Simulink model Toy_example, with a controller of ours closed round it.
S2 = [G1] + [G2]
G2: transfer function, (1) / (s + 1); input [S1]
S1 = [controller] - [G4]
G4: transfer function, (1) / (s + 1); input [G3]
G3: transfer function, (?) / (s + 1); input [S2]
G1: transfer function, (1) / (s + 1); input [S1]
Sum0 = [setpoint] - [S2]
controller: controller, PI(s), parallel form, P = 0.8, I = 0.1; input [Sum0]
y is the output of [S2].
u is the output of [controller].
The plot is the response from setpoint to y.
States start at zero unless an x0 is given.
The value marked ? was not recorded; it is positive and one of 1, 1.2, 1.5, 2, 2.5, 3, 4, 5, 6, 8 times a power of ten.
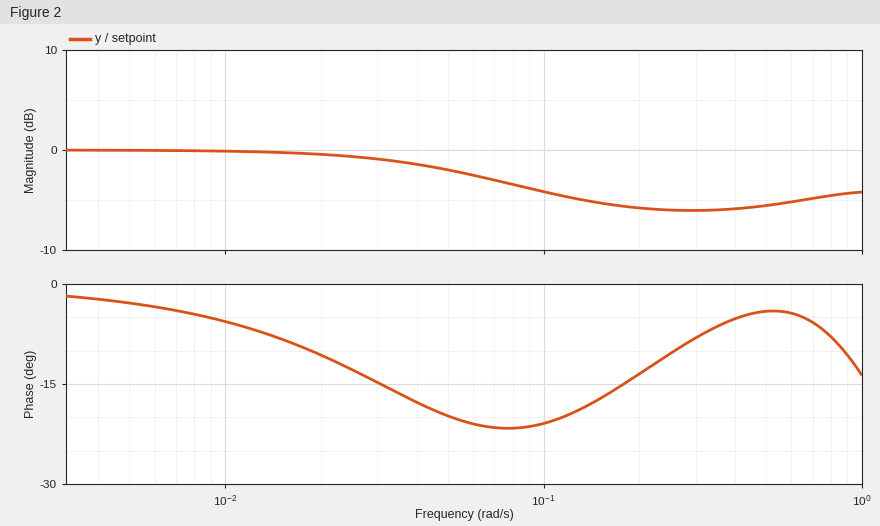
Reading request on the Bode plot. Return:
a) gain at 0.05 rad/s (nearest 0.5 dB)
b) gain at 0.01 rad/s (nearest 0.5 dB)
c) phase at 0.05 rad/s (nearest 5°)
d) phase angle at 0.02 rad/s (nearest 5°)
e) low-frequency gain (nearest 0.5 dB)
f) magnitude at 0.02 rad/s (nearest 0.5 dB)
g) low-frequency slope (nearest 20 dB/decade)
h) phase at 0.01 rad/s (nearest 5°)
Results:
-2.0 dB
0.0 dB
-20°
-10°
0.0 dB
-0.5 dB
0 dB/decade
-5°
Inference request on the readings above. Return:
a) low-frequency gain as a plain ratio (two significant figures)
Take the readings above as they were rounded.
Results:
1.0
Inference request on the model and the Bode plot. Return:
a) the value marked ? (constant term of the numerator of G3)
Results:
0.5
